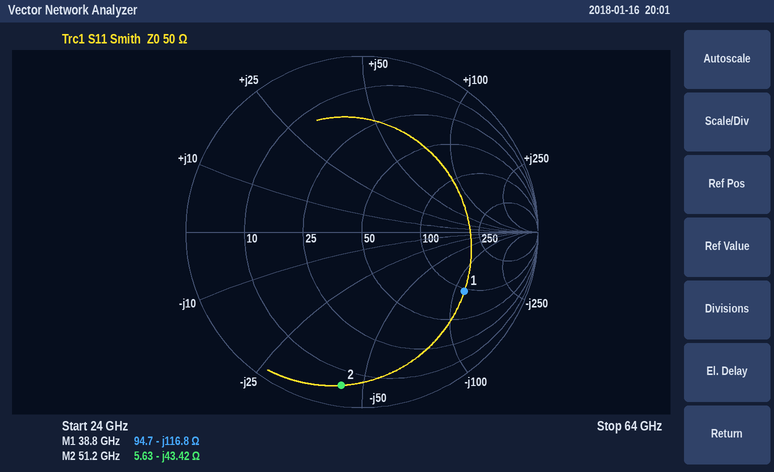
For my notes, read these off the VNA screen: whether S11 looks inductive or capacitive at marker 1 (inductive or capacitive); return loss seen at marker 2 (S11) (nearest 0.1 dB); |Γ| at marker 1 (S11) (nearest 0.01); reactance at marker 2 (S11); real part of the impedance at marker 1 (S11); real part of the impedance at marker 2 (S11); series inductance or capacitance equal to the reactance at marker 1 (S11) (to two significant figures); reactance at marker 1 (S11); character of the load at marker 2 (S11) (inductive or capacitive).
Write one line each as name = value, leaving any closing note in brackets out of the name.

whether S11 looks inductive or capacitive at marker 1 = capacitive
return loss seen at marker 2 (S11) = 1.1 dB
|Γ| at marker 1 (S11) = 0.67
reactance at marker 2 = -43.42 Ω
real part of the impedance at marker 1 = 94.7 Ω
real part of the impedance at marker 2 = 5.63 Ω
series inductance or capacitance equal to the reactance at marker 1 (S11) = 35 fF
reactance at marker 1 = -116.8 Ω
character of the load at marker 2 (S11) = capacitive
